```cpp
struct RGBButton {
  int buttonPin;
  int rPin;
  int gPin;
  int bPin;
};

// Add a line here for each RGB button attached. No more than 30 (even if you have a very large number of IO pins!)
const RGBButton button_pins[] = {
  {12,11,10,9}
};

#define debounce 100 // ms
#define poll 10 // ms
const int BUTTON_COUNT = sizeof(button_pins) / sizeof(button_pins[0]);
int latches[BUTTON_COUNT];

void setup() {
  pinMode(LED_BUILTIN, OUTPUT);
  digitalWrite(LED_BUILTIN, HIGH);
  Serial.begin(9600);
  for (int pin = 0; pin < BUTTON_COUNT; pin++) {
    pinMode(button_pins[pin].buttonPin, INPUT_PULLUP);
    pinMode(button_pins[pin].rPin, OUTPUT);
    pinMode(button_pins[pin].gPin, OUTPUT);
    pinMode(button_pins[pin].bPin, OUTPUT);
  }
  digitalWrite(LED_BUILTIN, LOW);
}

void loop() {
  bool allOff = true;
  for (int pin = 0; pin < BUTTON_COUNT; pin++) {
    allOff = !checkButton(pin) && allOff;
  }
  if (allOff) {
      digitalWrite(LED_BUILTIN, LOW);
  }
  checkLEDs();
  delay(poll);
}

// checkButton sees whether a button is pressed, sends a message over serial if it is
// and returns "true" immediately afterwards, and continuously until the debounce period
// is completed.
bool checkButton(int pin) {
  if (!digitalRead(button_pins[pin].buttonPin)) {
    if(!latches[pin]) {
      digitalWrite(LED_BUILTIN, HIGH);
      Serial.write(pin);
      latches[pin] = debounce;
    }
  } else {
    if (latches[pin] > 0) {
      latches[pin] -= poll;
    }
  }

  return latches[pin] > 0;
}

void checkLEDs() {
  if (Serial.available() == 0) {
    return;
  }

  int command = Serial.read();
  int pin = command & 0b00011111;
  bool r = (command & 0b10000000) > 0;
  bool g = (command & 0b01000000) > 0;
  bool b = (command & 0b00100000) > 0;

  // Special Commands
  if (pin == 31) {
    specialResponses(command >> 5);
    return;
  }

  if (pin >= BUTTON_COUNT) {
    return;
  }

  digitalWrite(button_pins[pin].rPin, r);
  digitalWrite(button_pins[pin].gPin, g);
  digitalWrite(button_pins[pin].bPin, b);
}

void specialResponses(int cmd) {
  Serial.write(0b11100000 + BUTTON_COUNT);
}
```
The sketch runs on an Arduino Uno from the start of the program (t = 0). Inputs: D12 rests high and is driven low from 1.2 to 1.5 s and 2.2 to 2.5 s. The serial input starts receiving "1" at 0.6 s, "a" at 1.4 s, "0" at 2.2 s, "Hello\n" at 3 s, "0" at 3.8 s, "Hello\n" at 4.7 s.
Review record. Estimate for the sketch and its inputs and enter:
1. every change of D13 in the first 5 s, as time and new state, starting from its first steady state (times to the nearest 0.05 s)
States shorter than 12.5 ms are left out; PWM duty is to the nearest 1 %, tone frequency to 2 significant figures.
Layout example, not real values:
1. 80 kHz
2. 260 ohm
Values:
1. 0 s low; 1.2 s high; 1.6 s low; 2.2 s high; 2.6 s low
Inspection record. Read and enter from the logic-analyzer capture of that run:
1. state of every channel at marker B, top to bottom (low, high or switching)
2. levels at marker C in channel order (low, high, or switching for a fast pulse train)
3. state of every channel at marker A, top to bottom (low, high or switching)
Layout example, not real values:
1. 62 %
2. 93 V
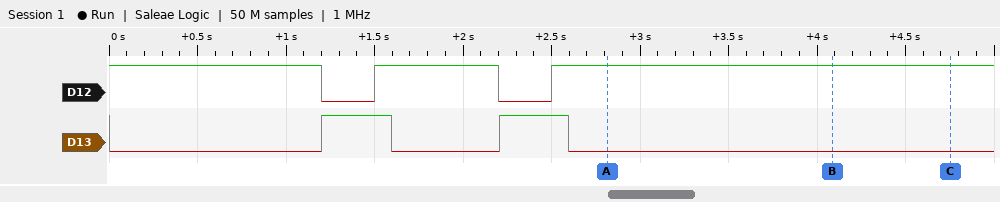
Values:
1. D12 high, D13 low
2. D12 high, D13 low
3. D12 high, D13 low
